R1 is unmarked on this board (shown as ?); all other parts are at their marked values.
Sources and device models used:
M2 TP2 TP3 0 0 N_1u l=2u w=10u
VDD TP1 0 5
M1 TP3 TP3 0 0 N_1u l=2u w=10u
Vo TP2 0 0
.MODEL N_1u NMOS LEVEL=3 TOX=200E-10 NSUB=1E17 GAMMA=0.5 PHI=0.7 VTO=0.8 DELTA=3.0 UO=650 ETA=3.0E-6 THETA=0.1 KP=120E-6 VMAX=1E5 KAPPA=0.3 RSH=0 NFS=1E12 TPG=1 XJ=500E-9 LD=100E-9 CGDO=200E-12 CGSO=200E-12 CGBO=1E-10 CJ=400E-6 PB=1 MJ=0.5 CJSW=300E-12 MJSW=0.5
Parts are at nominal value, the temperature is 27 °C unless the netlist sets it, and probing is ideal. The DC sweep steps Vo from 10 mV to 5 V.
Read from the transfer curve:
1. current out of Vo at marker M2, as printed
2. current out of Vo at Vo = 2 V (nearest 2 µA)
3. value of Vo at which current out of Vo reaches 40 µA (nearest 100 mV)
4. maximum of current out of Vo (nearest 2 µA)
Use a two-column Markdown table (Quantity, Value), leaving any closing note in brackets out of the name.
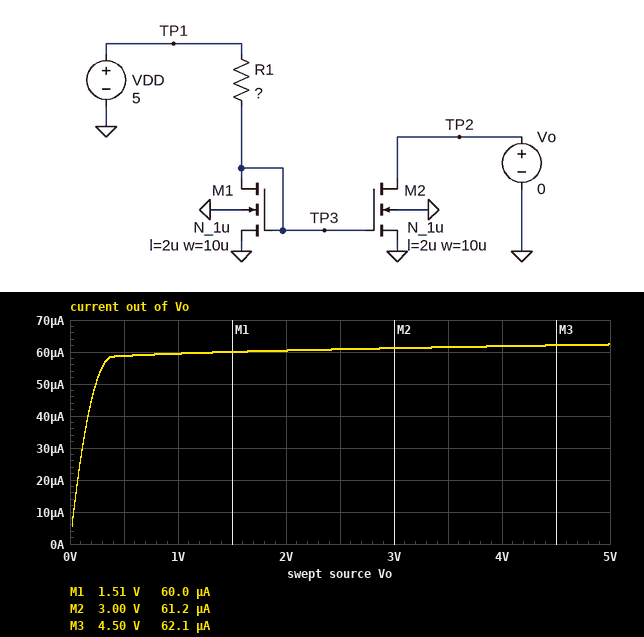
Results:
| Quantity | Value |
|---|---|
| current out of Vo at marker M2, as printed | 61.2 µA |
| current out of Vo at Vo = 2 V | 60 µA |
| value of Vo at which current out of Vo reaches 40 µA | 200 mV |
| maximum of current out of Vo | 62 µA |
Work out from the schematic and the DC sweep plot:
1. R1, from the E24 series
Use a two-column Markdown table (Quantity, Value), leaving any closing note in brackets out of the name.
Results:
| Quantity | Value |
|---|---|
| R1, from the E24 series | 62 kΩ |
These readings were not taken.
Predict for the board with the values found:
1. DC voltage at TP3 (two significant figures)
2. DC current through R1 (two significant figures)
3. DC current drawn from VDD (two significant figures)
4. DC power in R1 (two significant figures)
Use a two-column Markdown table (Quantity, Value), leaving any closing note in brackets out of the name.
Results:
| Quantity | Value |
|---|---|
| DC voltage at TP3 | 1.3 V |
| DC current through R1 | 60 µA |
| DC current drawn from VDD | 60 µA |
| DC power in R1 | 220 µW |
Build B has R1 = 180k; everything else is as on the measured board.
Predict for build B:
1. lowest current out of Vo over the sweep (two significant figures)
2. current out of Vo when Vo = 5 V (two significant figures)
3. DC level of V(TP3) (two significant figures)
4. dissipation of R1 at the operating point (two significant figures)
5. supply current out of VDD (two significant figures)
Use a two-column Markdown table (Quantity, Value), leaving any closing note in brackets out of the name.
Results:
| Quantity | Value |
|---|---|
| lowest current out of Vo over the sweep | 1.8 µA |
| current out of Vo when Vo = 5 V | 23 µA |
| DC level of V(TP3) | 1.1 V |
| dissipation of R1 at the operating point | 85 µW |
| supply current out of VDD | 22 µA |
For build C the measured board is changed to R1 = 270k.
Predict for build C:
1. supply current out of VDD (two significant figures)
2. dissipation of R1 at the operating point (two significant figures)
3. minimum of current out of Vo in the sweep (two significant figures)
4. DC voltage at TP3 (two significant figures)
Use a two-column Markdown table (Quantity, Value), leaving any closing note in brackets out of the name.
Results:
| Quantity | Value |
|---|---|
| supply current out of VDD | 15 µA |
| dissipation of R1 at the operating point | 58 µW |
| minimum of current out of Vo in the sweep | 1.5 µA |
| DC voltage at TP3 | 1.0 V |
